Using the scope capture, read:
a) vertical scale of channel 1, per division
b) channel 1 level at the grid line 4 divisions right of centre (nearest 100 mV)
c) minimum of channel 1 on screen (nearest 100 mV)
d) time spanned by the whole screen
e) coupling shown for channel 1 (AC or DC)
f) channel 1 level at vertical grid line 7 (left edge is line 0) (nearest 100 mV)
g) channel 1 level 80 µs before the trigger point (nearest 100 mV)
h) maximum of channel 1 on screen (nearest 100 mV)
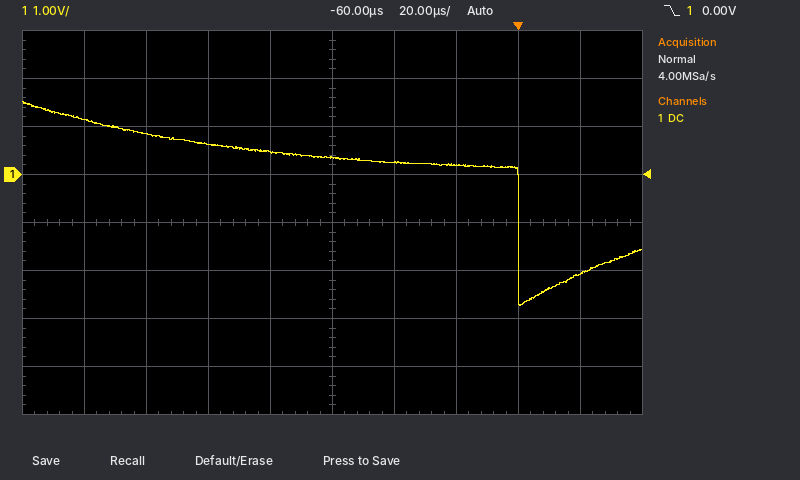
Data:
1 V
-2.1 V
-2.7 V
200 µs
DC
200 mV
500 mV
1.5 V
